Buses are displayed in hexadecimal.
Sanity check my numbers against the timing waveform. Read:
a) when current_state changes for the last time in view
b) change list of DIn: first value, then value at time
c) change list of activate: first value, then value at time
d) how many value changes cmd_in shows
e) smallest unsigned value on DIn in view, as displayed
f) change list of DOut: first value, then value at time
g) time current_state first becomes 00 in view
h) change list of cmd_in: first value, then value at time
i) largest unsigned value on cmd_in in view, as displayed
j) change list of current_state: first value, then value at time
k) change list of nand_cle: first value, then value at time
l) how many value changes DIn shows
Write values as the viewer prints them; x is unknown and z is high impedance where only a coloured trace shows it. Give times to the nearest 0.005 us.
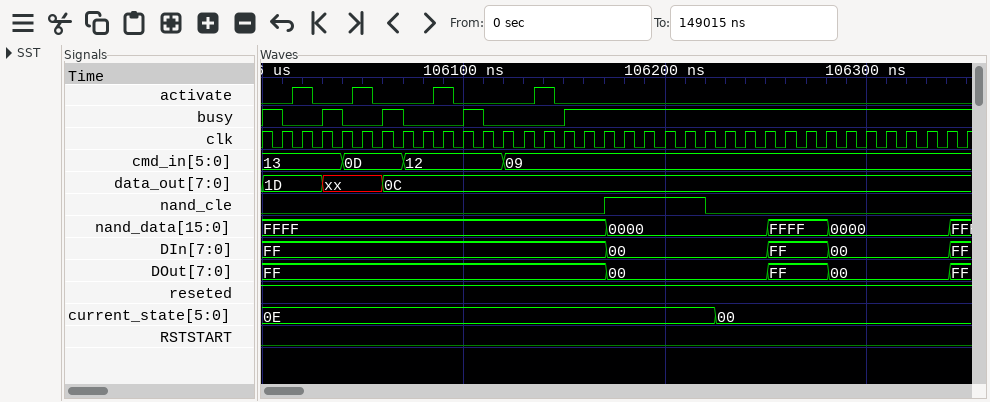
106.225 us
FF, 00 at 106.17 us, FF at 106.25 us, 00 at 106.28 us, FF at 106.34 us
0, 1 at 106.015 us, 0 at 106.025 us, 1 at 106.045 us, 0 at 106.055 us, 1 at 106.085 us, 0 at 106.095 us, 1 at 106.135 us, 0 at 106.145 us
3
00
FF, 00 at 106.17 us, FF at 106.25 us, 00 at 106.28 us, FF at 106.34 us
106.225 us
13, 0D at 106.04 us, 12 at 106.07 us, 09 at 106.12 us
13
0E, 00 at 106.225 us
0, 1 at 106.17 us, 0 at 106.22 us
4
